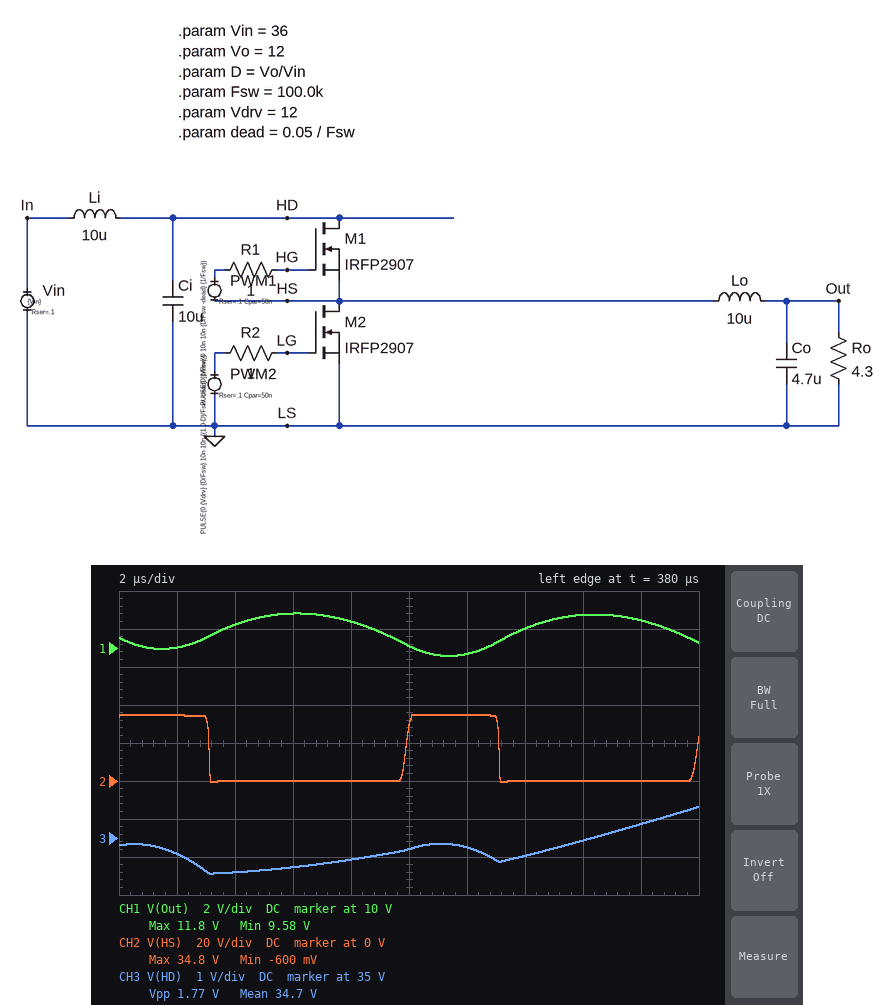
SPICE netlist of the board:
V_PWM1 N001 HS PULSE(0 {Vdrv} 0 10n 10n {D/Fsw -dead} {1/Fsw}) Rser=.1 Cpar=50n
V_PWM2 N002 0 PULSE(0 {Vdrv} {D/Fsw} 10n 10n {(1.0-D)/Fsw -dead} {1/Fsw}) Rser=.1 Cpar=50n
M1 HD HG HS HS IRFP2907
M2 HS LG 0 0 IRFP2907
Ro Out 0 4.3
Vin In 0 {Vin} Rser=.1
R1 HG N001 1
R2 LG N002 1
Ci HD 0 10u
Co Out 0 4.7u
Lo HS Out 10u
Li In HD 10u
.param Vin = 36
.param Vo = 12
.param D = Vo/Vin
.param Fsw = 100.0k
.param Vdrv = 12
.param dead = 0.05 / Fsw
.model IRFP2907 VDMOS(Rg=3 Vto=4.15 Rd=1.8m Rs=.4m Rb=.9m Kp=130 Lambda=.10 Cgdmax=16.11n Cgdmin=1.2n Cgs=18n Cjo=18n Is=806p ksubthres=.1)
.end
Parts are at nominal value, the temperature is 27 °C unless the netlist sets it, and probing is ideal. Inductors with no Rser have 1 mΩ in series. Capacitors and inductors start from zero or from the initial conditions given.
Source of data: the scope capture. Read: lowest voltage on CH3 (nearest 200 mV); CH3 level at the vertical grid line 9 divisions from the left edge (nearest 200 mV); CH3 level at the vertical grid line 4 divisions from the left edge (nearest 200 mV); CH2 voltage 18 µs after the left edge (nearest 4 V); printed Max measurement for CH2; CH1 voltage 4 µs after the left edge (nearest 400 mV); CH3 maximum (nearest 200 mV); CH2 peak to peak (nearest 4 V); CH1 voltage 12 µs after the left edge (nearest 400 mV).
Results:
34.0 V
35.4 V
34.4 V
0 V
34.8 V
11.2 V
35.8 V
36 V
9.6 V
